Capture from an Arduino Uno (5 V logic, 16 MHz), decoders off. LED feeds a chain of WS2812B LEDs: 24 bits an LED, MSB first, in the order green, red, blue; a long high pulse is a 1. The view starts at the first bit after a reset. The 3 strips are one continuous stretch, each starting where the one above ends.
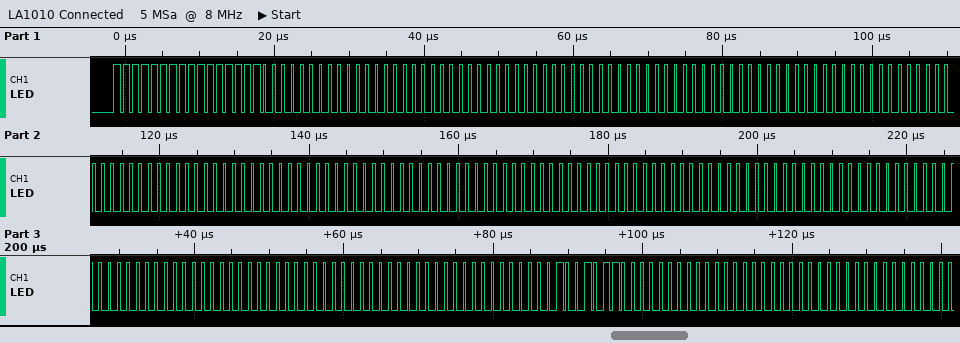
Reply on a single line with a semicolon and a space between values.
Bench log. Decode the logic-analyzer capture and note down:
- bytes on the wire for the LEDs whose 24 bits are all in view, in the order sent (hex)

FF FF 00 00 00 00 00 00 00 00 00 00 00 00 00 00 00 00 00 00 00 00 00 00 00 00 00 00 00 96 00 00 00
